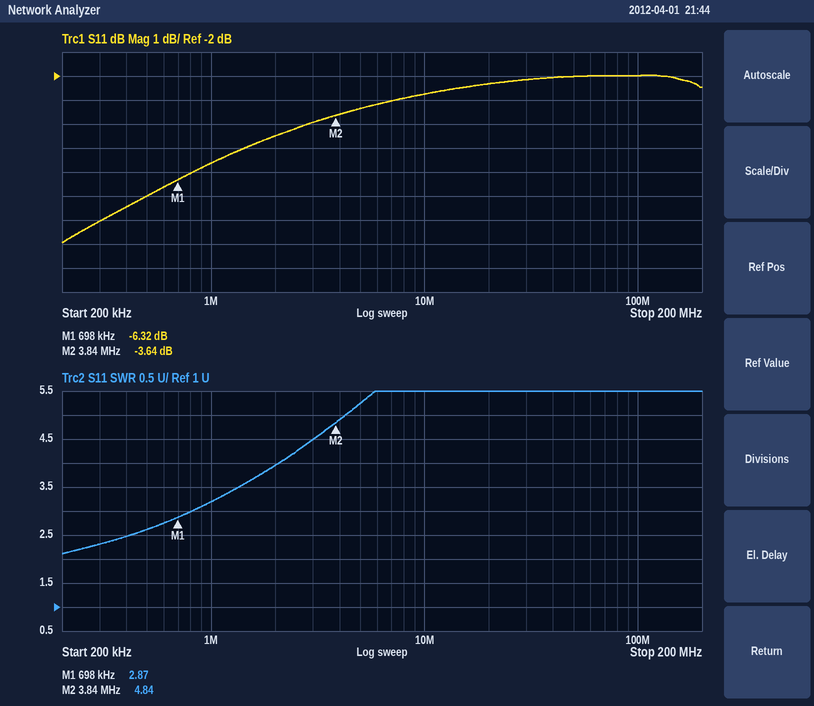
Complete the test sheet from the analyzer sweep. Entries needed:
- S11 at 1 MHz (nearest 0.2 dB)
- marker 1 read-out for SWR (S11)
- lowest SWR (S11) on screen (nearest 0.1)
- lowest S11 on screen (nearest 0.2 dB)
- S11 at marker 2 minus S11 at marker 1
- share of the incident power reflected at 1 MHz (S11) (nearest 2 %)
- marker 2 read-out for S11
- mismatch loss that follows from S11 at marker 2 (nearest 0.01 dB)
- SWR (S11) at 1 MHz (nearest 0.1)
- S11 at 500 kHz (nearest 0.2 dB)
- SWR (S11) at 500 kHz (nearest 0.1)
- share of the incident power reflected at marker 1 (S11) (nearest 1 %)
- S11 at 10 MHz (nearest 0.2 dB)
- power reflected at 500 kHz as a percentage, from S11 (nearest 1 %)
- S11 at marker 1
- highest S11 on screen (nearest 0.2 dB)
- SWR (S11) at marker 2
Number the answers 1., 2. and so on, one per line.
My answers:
1. -5.6 dB
2. 2.87
3. 2.1
4. -9.0 dB
5. 2.68 dB
6. 28 %
7. -3.64 dB
8. 2.46 dB
9. 3.2
10. -7.0 dB
11. 2.6
12. 23 %
13. -2.8 dB
14. 20 %
15. -6.32 dB
16. -2.0 dB
17. 4.84
